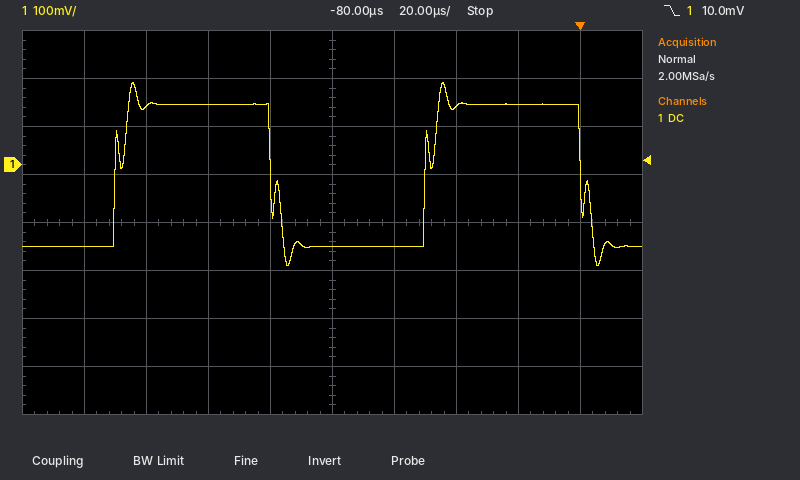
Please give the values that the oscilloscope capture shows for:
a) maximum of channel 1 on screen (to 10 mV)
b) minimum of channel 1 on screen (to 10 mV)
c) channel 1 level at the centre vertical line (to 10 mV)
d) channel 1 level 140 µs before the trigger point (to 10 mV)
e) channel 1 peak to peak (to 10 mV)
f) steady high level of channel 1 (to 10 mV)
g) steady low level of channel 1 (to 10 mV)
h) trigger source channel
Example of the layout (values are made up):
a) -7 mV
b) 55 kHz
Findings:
a) 170 mV
b) -210 mV
c) -170 mV
d) 120 mV
e) 380 mV
f) 130 mV
g) -170 mV
h) channel 1
